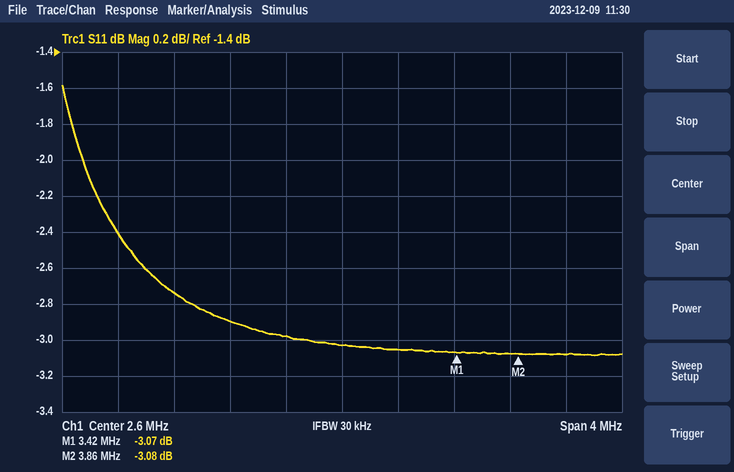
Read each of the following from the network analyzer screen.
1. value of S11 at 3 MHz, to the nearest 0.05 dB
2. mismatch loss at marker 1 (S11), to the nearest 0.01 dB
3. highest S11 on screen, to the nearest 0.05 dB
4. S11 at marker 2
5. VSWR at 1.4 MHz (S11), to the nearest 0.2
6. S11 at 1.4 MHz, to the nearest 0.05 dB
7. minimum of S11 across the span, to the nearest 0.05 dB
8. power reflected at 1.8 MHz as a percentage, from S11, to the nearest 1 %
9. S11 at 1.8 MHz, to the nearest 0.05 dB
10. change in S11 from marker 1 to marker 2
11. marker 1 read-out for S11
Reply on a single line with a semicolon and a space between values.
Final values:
-3.05 dB; 2.95 dB; -1.60 dB; -3.08 dB; 6.4; -2.75 dB; -3.10 dB; 51 %; -2.90 dB; -0.01 dB; -3.07 dB
